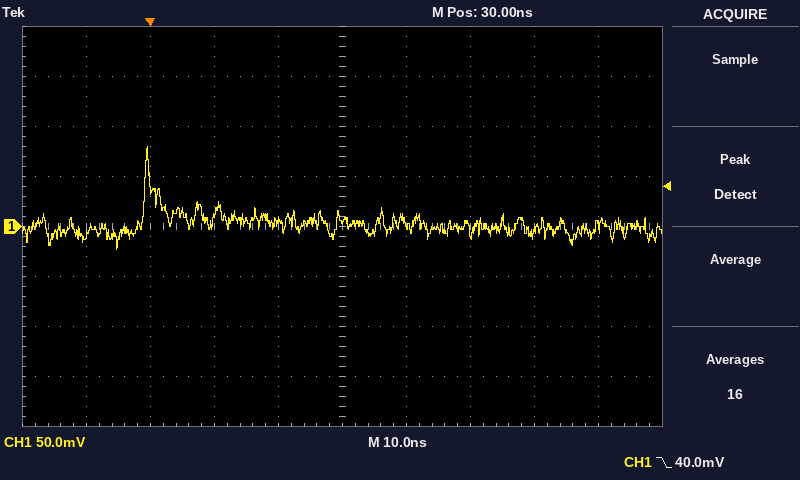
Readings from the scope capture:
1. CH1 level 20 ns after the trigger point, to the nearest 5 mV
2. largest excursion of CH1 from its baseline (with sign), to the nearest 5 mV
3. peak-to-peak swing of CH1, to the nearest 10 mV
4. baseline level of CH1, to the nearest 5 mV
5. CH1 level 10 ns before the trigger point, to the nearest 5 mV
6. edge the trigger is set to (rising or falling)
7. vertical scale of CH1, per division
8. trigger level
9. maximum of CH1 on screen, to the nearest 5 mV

5 mV
+80 mV
100 mV
0 mV
-10 mV
falling
50 mV
40.0 mV
80 mV
